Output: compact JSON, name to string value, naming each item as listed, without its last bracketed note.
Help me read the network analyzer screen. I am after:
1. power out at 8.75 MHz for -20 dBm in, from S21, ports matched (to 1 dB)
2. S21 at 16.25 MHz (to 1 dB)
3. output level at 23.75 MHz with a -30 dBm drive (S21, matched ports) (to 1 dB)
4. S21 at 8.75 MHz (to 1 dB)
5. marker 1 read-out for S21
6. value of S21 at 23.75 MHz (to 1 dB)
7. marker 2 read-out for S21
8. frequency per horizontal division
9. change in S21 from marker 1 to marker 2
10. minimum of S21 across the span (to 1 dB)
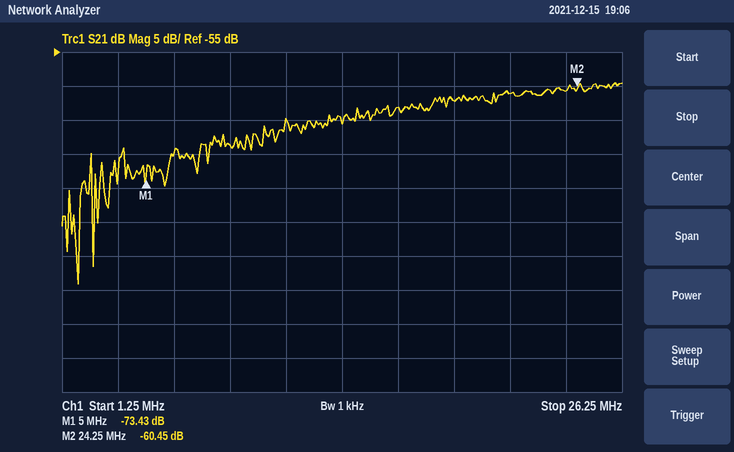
{"power out at 8.75 MHz for -20 dBm in, from S21, ports matched": "-89 dBm", "S21 at 16.25 MHz": "-63 dB", "output level at 23.75 MHz with a -30 dBm drive (S21, matched ports)": "-91 dBm", "S21 at 8.75 MHz": "-69 dB", "marker 1 read-out for S21": "-73.43 dB", "value of S21 at 23.75 MHz": "-61 dB", "marker 2 read-out for S21": "-60.45 dB", "frequency per horizontal division": "2.5 MHz", "change in S21 from marker 1 to marker 2": "12.98 dB", "minimum of S21 across the span": "-89 dB"}
